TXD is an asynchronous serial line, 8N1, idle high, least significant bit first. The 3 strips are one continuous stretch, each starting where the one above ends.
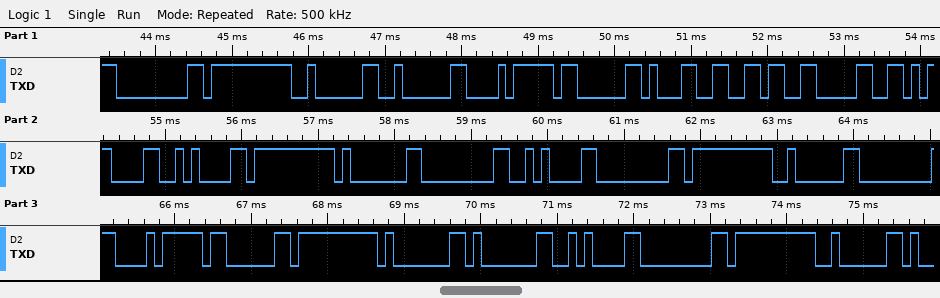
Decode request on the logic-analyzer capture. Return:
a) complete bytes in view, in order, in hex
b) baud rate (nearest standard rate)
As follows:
00 FF 02 02 E8 03 31 36 30 0D 0A FF 01 00 0A 00 FF 02 00 E8 03 FF 01 01 0A 00 FF 02
9600 baud
